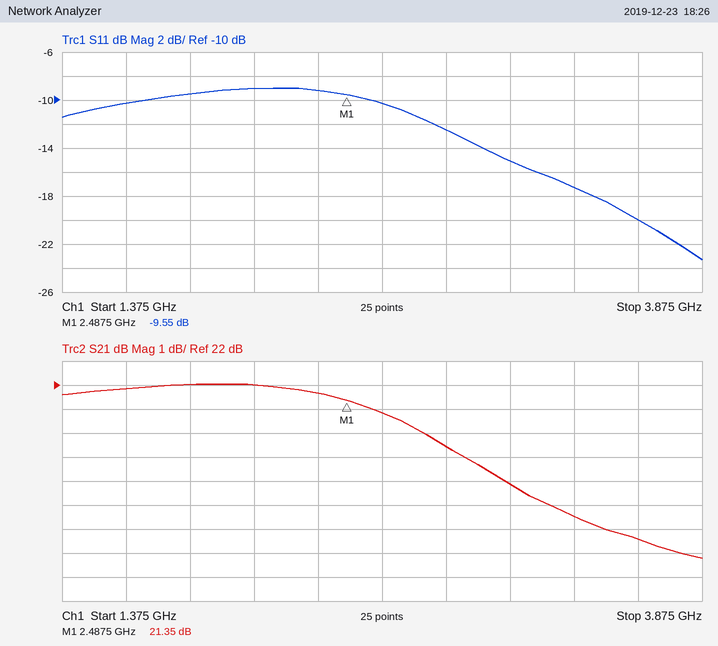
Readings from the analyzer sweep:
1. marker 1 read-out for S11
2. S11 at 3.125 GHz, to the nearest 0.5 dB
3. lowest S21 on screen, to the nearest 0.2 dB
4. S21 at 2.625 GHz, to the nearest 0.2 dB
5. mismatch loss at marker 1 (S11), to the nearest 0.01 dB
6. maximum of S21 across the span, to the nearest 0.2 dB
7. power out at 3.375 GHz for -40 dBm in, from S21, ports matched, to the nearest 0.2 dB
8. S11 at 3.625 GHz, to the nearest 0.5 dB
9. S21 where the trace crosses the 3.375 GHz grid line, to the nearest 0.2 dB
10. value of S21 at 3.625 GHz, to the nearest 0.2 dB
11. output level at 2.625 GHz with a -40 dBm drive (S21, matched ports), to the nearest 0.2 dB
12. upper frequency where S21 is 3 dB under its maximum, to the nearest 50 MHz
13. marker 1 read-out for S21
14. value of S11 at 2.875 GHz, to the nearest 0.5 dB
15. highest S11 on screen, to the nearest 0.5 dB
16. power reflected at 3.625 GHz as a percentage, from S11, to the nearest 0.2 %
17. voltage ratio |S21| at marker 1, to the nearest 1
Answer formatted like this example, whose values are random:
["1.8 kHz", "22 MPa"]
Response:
["-9.55 dB", "-15.0 dB", "14.8 dB", "20.8 dB", "0.51 dB", "22.0 dB", "-23.4 dBm", "-20.0 dB", "16.6 dB", "15.6 dB", "-19.2 dBm", "2.95 GHz", "21.35 dB", "-12.5 dB", "-9.0 dB", "1.0 %", "12"]
